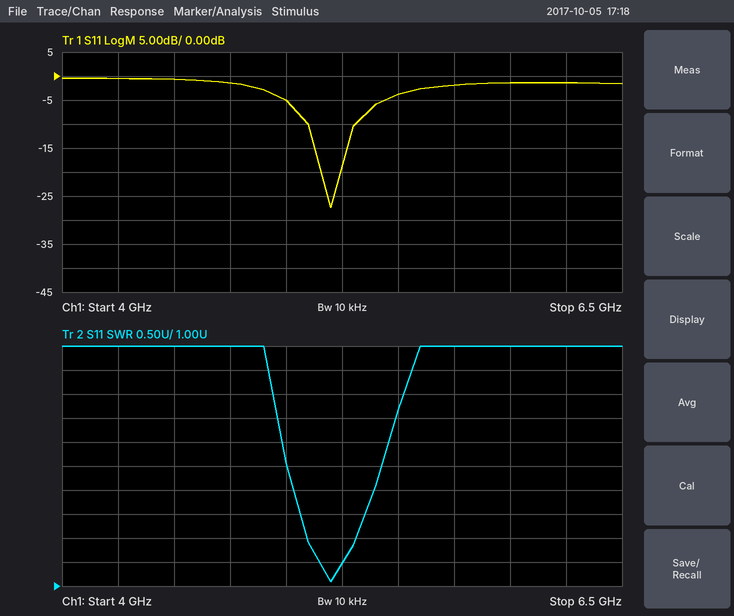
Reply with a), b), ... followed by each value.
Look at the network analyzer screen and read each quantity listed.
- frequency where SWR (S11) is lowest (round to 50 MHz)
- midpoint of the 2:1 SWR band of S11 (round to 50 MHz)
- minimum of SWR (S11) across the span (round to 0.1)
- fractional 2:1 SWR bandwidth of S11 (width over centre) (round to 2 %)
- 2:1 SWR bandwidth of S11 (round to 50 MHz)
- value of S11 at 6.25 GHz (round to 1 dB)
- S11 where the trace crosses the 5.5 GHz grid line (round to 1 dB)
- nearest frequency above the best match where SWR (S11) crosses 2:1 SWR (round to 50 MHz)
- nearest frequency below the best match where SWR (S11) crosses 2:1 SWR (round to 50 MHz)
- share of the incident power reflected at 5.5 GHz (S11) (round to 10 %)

a) 5.20 GHz
b) 5.20 GHz
c) 1.1
d) 4 %
e) 200 MHz
f) -1 dB
g) -4 dB
h) 5.30 GHz
i) 5.10 GHz
j) 40 %
